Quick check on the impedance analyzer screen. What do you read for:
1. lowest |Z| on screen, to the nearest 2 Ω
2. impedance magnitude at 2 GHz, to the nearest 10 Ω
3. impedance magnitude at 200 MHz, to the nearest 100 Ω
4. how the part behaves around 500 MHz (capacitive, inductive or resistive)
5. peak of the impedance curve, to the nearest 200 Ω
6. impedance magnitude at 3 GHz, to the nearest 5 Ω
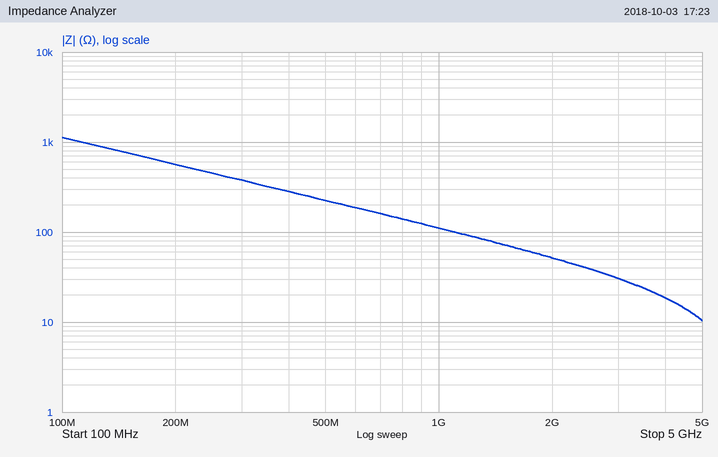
10 Ω
50 Ω
600 Ω
capacitive
1.2 kΩ
30 Ω
